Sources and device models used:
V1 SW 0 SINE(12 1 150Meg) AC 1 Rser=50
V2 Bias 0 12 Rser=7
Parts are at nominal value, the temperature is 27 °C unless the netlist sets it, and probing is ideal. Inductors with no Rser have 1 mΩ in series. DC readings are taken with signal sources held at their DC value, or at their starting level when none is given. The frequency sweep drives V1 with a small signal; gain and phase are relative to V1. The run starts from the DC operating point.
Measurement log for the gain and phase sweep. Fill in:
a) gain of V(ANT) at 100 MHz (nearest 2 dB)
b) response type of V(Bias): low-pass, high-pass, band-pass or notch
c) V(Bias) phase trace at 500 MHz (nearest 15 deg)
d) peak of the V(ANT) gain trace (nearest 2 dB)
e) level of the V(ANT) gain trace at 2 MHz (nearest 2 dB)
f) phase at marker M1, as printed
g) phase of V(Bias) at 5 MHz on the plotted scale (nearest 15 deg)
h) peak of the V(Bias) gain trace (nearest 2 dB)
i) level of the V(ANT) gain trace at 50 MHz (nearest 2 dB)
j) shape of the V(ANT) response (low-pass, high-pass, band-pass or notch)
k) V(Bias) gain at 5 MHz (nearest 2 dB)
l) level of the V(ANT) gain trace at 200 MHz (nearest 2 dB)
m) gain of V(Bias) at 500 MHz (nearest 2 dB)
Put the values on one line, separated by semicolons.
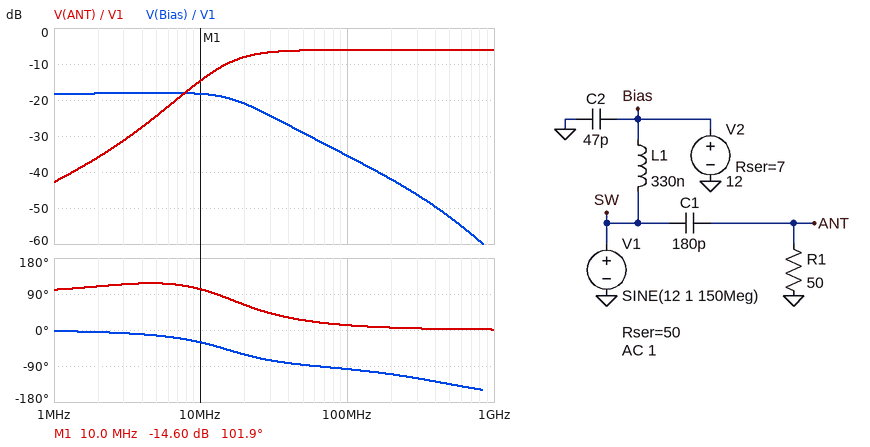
-6 dB; low-pass; -135 deg; -6 dB; -36 dB; 101.9 deg; -15 deg; -18 dB; -6 dB; high-pass; -18 dB; -6 dB; -52 dB
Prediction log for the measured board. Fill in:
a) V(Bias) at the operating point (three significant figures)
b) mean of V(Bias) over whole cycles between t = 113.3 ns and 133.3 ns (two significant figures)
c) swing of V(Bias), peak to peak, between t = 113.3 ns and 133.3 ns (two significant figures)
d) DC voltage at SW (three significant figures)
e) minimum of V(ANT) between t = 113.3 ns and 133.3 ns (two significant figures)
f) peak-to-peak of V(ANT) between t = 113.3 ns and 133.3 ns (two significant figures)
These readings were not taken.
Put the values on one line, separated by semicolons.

12.0 V; 12 V; 22 mV; 12.0 V; -500 mV; 1.0 V
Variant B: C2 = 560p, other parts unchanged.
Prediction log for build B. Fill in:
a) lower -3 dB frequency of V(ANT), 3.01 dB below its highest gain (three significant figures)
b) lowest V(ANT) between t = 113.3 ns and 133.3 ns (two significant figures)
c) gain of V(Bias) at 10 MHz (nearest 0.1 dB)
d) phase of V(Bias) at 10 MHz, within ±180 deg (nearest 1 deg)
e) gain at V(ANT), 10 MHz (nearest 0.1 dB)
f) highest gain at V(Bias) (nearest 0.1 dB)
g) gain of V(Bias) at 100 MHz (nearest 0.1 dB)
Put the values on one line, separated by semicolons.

17.4 MHz; -500 mV; -18.4 dB; -42 deg; -15.1 dB; -18.2 dB; -43.7 dB
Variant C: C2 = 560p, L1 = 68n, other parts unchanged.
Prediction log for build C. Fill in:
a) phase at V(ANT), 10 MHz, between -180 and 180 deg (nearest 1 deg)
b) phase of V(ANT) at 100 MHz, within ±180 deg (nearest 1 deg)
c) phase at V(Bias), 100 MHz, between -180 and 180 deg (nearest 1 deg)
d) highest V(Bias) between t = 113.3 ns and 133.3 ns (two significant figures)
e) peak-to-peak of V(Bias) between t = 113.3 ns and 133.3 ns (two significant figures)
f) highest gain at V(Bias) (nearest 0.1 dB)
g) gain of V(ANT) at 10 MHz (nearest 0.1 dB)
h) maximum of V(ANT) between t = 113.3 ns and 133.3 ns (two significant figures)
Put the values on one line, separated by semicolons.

76 deg; 38 deg; -128 deg; 12 V; 28 mV; -18.2 dB; -24.3 dB; 470 mV
